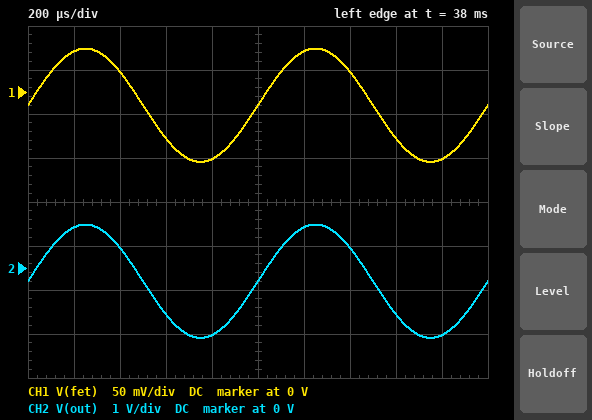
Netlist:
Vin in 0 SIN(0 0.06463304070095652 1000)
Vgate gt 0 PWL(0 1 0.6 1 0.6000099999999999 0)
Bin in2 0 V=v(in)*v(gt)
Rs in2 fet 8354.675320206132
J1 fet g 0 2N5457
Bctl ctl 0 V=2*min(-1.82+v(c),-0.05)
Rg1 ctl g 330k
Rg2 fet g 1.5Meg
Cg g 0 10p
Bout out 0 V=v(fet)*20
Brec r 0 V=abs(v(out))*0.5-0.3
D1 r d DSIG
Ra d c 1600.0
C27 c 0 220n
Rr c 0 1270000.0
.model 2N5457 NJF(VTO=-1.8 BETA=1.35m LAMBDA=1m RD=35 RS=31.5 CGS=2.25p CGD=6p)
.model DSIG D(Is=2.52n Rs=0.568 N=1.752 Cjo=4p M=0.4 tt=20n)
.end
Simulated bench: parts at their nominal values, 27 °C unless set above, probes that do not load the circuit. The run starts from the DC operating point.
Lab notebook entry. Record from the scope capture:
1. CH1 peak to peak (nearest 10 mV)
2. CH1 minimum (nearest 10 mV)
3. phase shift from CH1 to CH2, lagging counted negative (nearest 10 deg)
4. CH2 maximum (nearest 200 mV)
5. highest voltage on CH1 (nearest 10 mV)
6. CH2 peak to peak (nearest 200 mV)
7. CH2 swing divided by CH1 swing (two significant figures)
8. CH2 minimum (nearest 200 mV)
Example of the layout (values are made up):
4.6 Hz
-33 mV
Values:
130 mV
-80 mV
0 deg
1.0 V
50 mV
2.6 V
20
-1.6 V
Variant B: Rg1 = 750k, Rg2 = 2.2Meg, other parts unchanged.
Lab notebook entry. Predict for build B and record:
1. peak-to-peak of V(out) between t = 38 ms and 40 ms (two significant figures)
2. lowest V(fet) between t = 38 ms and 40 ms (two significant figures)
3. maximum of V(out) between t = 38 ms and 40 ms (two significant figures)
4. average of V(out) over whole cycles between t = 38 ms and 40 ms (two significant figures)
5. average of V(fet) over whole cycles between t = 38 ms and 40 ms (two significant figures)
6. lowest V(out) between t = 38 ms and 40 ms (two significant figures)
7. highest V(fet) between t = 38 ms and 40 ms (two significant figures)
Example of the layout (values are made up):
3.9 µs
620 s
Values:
2.6 V
-74 mV
1.1 V
-190 mV
-9.6 mV
-1.5 V
55 mV
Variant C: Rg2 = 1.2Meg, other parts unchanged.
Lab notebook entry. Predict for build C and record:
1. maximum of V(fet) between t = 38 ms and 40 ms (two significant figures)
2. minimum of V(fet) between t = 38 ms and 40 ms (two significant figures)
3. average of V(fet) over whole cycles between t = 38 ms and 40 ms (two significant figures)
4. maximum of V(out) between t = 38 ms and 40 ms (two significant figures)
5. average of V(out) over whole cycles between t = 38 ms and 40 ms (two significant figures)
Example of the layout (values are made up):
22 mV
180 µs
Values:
47 mV
-82 mV
-18 mV
930 mV
-350 mV
